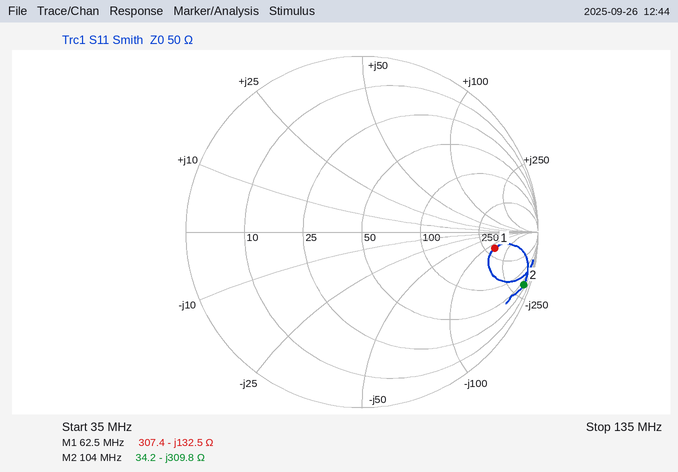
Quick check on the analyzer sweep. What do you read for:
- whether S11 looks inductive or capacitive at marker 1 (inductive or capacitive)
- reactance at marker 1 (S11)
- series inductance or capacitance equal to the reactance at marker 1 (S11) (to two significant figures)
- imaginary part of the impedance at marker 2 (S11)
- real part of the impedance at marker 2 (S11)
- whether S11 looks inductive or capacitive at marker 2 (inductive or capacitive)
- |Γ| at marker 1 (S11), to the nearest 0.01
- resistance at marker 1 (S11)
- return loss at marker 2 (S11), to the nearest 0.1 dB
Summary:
capacitive
-132.5 Ω
19 pF
-309.8 Ω
34.2 Ω
capacitive
0.76
307.4 Ω
0.3 dB
